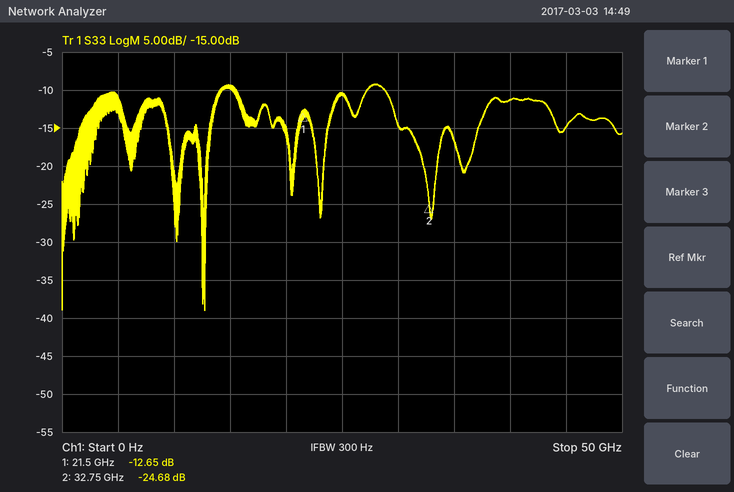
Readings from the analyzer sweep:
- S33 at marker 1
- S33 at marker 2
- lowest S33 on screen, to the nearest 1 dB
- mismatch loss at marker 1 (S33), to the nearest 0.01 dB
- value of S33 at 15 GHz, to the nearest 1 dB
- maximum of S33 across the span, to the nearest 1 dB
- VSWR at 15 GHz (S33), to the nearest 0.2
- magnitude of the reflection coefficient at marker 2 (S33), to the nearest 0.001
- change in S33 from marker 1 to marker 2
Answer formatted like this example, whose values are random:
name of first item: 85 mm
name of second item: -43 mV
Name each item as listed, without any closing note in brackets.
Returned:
S33 at marker 1: -12.65 dB
S33 at marker 2: -24.68 dB
lowest S33 on screen, to the nearest 1 dB: -39 dB
mismatch loss at marker 1 (S33), to the nearest 0.01 dB: 0.24 dB
value of S33 at 15 GHz, to the nearest 1 dB: -10 dB
maximum of S33 across the span, to the nearest 1 dB: -9 dB
VSWR at 15 GHz (S33), to the nearest 0.2: 2.0
magnitude of the reflection coefficient at marker 2 (S33), to the nearest 0.001: 0.058
change in S33 from marker 1 to marker 2: -12.03 dB
